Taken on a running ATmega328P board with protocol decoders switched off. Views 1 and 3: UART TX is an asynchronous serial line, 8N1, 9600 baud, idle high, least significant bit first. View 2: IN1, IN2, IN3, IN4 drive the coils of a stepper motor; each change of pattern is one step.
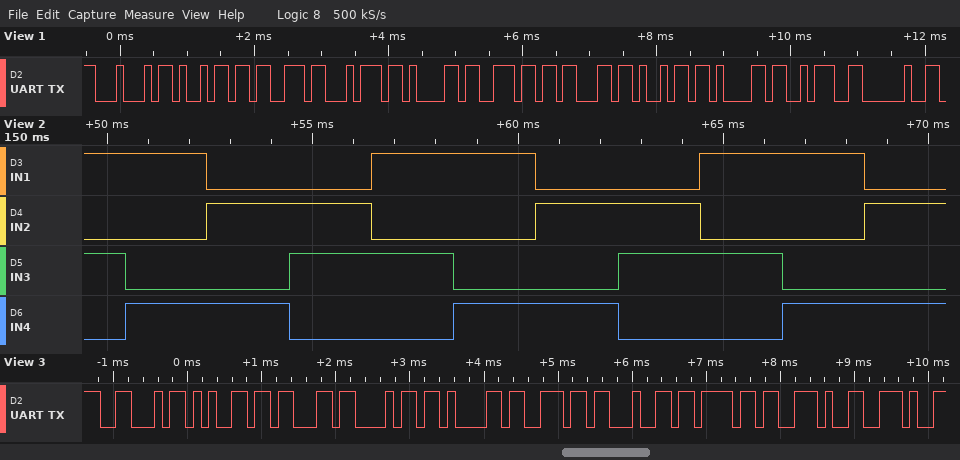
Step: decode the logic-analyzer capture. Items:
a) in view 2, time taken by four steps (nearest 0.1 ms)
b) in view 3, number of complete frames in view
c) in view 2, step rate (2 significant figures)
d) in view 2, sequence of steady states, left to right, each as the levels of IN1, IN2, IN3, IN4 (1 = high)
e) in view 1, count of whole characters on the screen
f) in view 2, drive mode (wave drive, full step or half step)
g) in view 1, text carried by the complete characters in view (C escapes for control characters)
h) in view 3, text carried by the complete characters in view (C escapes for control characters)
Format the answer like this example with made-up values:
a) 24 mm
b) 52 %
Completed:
a) 8.0 ms
b) 10
c) 500 steps/s
d) 1010 1001 0101 0110 1010 1001 0101 0110 1010 1001 0101
e) 11
f) full step
g) "Distancia: "
h) "Fechando.."
